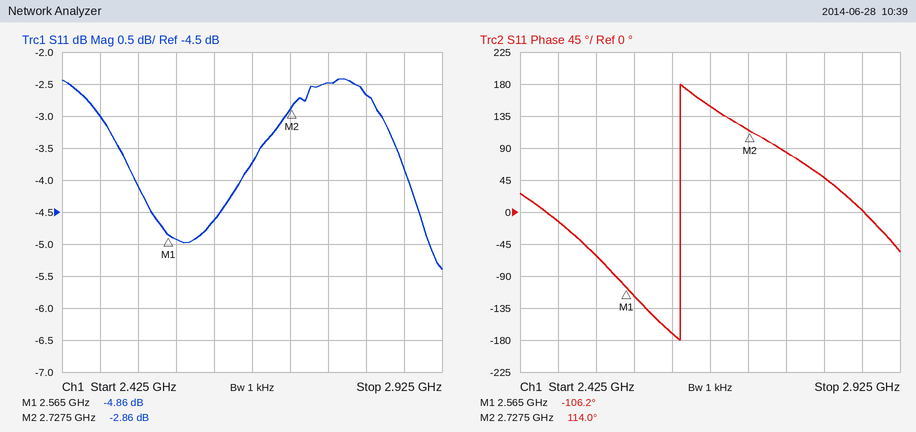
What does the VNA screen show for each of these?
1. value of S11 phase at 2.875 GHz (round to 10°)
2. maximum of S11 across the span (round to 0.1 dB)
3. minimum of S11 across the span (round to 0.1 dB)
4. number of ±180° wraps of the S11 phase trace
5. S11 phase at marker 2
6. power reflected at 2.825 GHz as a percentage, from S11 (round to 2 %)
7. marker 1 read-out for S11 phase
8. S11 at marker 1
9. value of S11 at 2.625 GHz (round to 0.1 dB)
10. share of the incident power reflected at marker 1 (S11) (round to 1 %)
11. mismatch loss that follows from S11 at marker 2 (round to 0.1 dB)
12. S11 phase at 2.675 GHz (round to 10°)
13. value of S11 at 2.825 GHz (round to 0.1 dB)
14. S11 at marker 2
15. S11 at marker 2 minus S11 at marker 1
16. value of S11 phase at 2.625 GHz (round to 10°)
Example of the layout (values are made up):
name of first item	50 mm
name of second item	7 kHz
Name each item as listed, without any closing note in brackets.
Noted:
value of S11 phase at 2.875 GHz	0°
maximum of S11 across the span	-2.4 dB
minimum of S11 across the span	-5.4 dB
number of ±180° wraps of the S11 phase trace	1
S11 phase at marker 2	114.0°
power reflected at 2.825 GHz as a percentage, from S11	54 %
marker 1 read-out for S11 phase	-106.2°
S11 at marker 1	-4.86 dB
value of S11 at 2.625 GHz	-4.6 dB
share of the incident power reflected at marker 1 (S11)	33 %
mismatch loss that follows from S11 at marker 2	3.2 dB
S11 phase at 2.675 GHz	150°
value of S11 at 2.825 GHz	-2.7 dB
S11 at marker 2	-2.86 dB
S11 at marker 2 minus S11 at marker 1	2.00 dB
value of S11 phase at 2.625 GHz	-170°
